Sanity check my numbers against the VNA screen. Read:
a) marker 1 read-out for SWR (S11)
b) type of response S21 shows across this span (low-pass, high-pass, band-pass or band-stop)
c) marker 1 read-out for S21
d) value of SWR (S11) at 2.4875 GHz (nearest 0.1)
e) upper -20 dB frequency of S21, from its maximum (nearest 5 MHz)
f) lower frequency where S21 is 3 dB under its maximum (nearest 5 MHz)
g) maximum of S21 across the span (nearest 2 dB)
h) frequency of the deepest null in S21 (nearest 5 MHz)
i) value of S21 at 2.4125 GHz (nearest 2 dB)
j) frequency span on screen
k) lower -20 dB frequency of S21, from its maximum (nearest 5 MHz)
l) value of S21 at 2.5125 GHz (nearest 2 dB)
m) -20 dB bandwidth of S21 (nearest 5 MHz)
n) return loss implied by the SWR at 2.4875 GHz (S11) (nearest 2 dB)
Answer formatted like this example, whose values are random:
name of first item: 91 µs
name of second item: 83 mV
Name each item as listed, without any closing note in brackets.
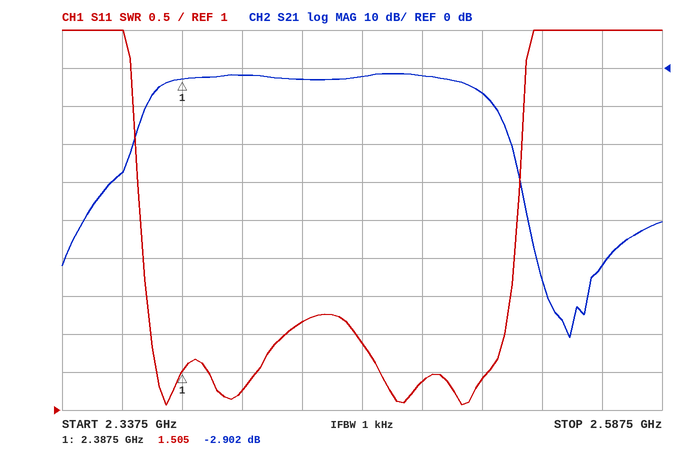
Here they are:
marker 1 read-out for SWR: 1.505
type of response S21 shows across this span: band-pass
marker 1 read-out for S21: -2.902 dB
value of SWR (S11) at 2.4875 GHz: 1.4
upper -20 dB frequency of S21, from its maximum: 2.525 GHz
lower frequency where S21 is 3 dB under its maximum: 2.380 GHz
maximum of S21 across the span: -2 dB
frequency of the deepest null in S21: 2.550 GHz
value of S21 at 2.4125 GHz: -2 dB
frequency span on screen: 250 MHz
lower -20 dB frequency of S21, from its maximum: 2.365 GHz
value of S21 at 2.5125 GHz: -6 dB
-20 dB bandwidth of S21: 160 MHz
return loss implied by the SWR at 2.4875 GHz (S11): 16 dB
